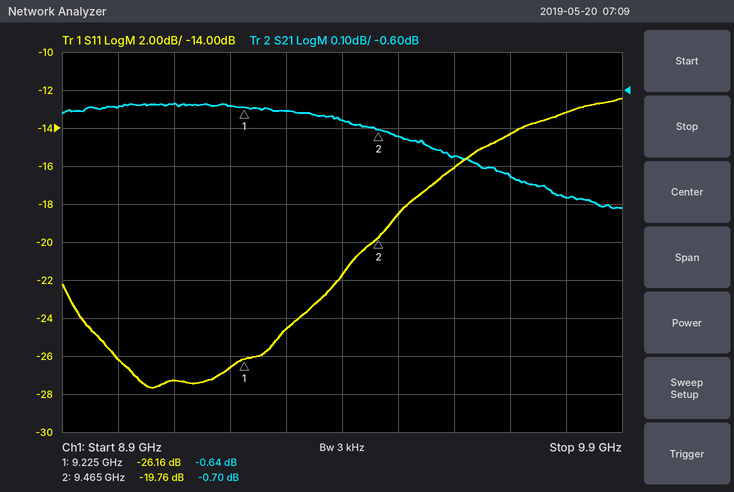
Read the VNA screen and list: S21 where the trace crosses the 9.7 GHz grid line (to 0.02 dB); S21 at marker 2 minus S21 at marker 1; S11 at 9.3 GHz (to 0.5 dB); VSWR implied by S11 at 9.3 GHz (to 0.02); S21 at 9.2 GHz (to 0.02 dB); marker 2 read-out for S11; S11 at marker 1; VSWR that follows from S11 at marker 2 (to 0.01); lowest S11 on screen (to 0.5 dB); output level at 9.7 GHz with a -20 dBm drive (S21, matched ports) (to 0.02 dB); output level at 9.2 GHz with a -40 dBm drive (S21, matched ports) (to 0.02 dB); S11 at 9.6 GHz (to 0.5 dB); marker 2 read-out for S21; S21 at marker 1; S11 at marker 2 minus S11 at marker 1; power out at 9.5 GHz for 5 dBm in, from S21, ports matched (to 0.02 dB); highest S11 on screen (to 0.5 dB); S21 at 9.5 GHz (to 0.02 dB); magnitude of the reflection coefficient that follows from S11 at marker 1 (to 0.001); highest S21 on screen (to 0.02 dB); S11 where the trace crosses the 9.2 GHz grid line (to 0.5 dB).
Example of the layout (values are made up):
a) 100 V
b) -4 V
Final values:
a) -0.82 dB
b) -0.06 dB
c) -24.5 dB
d) 1.12
e) -0.64 dB
f) -19.76 dB
g) -26.16 dB
h) 1.23
i) -27.5 dB
j) -20.82 dBm
k) -40.64 dBm
l) -16.0 dB
m) -0.70 dB
n) -0.64 dB
o) 6.40 dB
p) 4.28 dBm
q) -12.5 dB
r) -0.72 dB
s) 0.049
t) -0.64 dB
u) -26.5 dB
